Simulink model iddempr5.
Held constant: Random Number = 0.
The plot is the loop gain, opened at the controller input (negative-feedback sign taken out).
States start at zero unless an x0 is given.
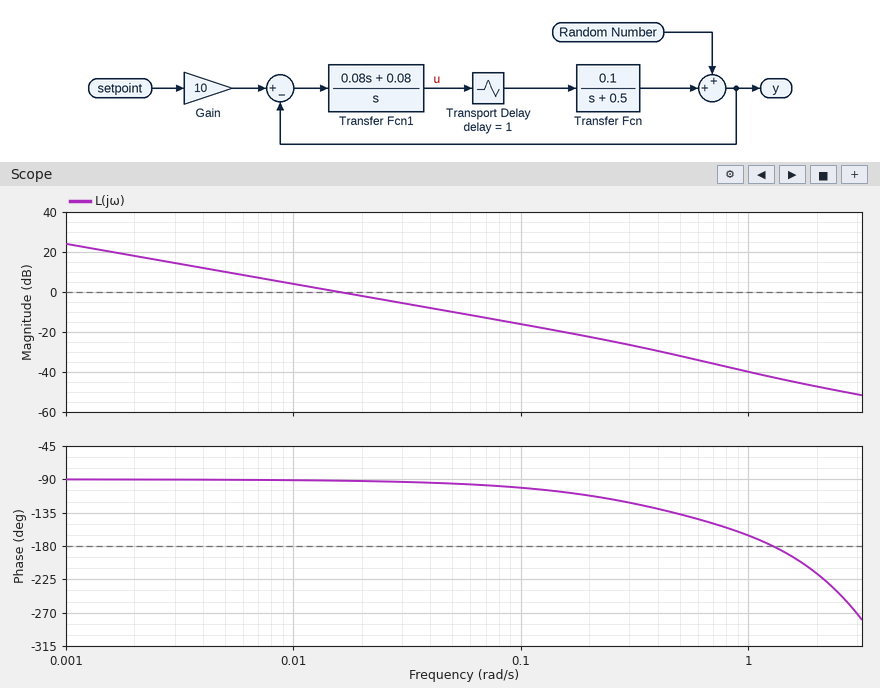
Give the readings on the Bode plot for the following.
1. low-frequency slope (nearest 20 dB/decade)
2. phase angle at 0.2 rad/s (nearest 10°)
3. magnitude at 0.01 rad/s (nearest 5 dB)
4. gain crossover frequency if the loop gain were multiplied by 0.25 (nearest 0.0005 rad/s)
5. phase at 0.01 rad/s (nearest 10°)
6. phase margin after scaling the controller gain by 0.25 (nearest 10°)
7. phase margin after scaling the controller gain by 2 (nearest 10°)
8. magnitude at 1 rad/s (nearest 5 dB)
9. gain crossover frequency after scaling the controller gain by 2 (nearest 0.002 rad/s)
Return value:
-20 dB/decade
-110°
5 dB
0.0040 rad/s
-90°
90°
90°
-40 dB
0.032 rad/s
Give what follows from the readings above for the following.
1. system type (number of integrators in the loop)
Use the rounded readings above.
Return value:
1
